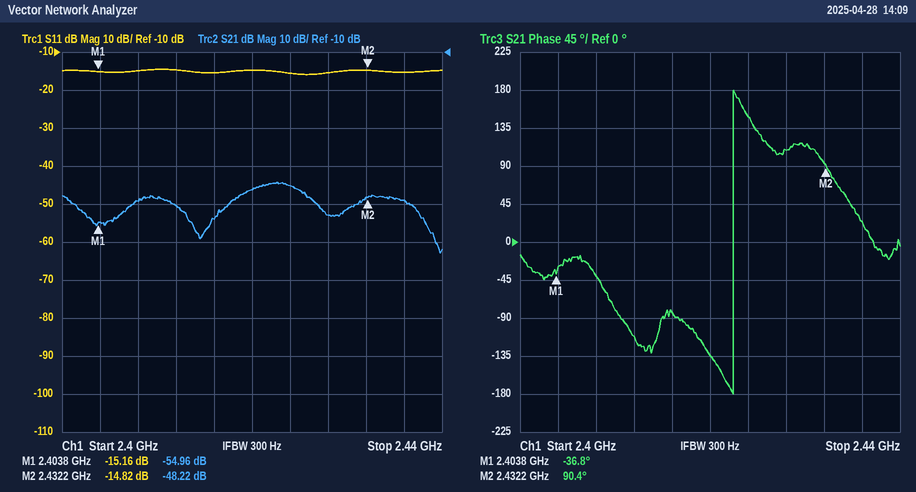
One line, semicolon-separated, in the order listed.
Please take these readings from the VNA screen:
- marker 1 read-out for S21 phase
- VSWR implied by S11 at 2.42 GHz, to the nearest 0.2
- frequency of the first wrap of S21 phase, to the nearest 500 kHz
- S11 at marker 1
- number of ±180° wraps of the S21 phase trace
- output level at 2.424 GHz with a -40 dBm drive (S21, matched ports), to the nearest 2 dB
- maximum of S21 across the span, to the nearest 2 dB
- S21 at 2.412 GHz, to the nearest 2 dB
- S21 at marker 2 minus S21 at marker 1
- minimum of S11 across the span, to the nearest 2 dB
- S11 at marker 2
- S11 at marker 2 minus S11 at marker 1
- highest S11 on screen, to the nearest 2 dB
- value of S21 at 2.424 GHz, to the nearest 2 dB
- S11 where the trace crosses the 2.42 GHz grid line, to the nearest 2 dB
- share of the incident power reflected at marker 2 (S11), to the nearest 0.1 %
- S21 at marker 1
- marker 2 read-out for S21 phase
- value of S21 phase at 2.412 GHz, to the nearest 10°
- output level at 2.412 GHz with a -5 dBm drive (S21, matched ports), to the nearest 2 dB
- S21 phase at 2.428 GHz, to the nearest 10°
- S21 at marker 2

-36.8°; 1.4; 2.4225 GHz; -15.16 dB; 1; -86 dBm; -44 dB; -50 dB; 6.74 dB; -16 dB; -14.82 dB; 0.34 dB; -14 dB; -46 dB; -14 dB; 3.3 %; -54.96 dB; 90.4°; -110°; -56 dBm; 110°; -48.22 dB
